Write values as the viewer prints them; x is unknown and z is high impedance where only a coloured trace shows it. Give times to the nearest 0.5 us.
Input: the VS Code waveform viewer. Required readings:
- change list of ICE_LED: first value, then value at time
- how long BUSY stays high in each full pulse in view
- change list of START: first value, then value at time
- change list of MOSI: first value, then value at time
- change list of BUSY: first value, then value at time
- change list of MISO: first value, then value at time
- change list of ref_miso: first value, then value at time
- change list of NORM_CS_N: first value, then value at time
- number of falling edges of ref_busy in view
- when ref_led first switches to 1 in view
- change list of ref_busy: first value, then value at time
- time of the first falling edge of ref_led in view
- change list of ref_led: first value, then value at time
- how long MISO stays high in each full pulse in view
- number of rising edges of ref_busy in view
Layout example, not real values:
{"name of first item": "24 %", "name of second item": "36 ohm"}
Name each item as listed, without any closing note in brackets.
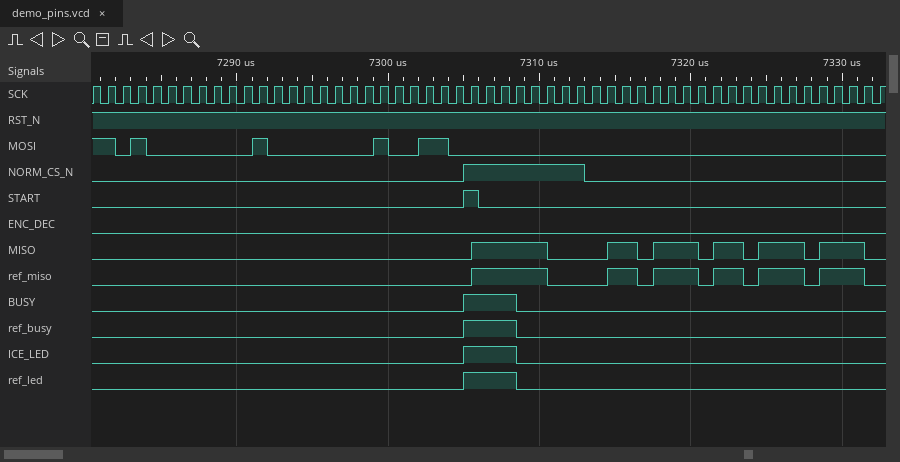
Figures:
{"change list of ICE_LED: first value, then value at time": "0, 1 at 7305 us, 0 at 7308.5 us", "how long BUSY stays high in each full pulse in view": "3.5 us", "change list of START: first value, then value at time": "0, 1 at 7305 us, 0 at 7306 us", "change list of MOSI: first value, then value at time": "1, 0 at 7282 us, 1 at 7283 us, 0 at 7284 us, 1 at 7291 us, 0 at 7292 us, 1 at 7299 us, 0 at 7300 us, 1 at 7302 us, 0 at 7304 us", "change list of BUSY: first value, then value at time": "0, 1 at 7305 us, 0 at 7308.5 us", "change list of MISO: first value, then value at time": "0, 1 at 7305.5 us, 0 at 7310.5 us, 1 at 7314.5 us, 0 at 7316.5 us, 1 at 7317.5 us, 0 at 7320.5 us, 1 at 7321.5 us, 0 at 7323.5 us, 1 at 7324.5 us, 0 at 7327.5 us, 1 at 7328.5 us, 0 at 7331.5 us", "change list of ref_miso: first value, then value at time": "0, 1 at 7305.5 us, 0 at 7310.5 us, 1 at 7314.5 us, 0 at 7316.5 us, 1 at 7317.5 us, 0 at 7320.5 us, 1 at 7321.5 us, 0 at 7323.5 us, 1 at 7324.5 us, 0 at 7327.5 us, 1 at 7328.5 us, 0 at 7331.5 us", "change list of NORM_CS_N: first value, then value at time": "0, 1 at 7305 us, 0 at 7313 us", "number of falling edges of ref_busy in view": "1", "when ref_led first switches to 1 in view": "7305 us", "change list of ref_busy: first value, then value at time": "0, 1 at 7305 us, 0 at 7308.5 us", "time of the first falling edge of ref_led in view": "7308.5 us", "change list of ref_led: first value, then value at time": "0, 1 at 7305 us, 0 at 7308.5 us", "how long MISO stays high in each full pulse in view": "5 us, 2 us, 3 us, 2 us, 3 us, 3 us", "number of rising edges of ref_busy in view": "1"}
